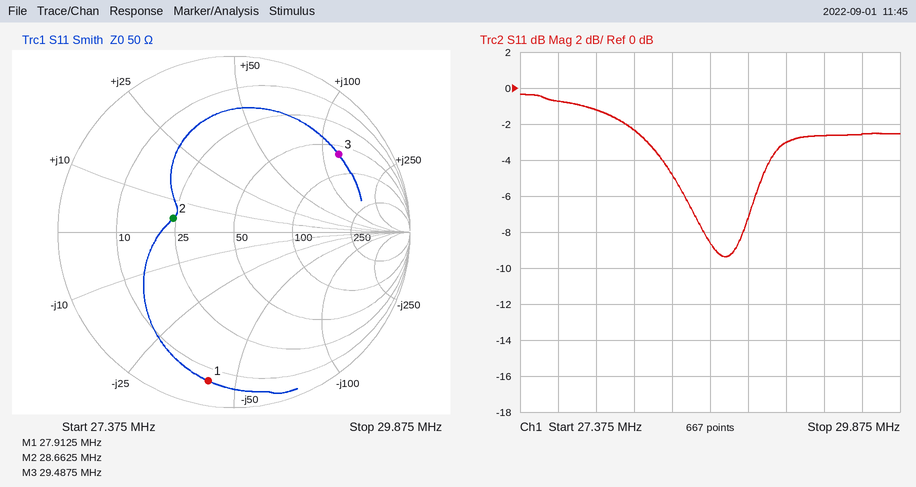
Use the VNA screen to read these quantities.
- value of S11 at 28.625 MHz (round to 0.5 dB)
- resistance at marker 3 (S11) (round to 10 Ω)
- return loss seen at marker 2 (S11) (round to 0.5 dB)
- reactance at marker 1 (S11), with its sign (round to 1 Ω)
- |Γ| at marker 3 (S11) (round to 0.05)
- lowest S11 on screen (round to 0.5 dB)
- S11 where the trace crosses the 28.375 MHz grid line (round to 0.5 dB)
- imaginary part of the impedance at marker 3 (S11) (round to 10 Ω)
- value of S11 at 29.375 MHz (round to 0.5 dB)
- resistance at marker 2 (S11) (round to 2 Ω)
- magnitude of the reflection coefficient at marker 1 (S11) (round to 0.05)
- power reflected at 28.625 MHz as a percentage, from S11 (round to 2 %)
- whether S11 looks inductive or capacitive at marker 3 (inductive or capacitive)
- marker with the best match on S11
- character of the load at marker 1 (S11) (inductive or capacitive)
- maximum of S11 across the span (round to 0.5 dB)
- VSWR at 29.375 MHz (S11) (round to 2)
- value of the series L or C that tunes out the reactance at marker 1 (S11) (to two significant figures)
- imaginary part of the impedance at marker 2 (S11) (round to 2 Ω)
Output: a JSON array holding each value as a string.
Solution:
["-8.5 dB", "60 Ω", "9.0 dB", "-42 Ω", "0.75", "-9.5 dB", "-5.0 dB", "+120 Ω", "-2.5 dB", "24 Ω", "0.85", "14 %", "inductive", "marker 2", "capacitive", "-0.5 dB", "6", "240 nH", "+4 Ω"]
